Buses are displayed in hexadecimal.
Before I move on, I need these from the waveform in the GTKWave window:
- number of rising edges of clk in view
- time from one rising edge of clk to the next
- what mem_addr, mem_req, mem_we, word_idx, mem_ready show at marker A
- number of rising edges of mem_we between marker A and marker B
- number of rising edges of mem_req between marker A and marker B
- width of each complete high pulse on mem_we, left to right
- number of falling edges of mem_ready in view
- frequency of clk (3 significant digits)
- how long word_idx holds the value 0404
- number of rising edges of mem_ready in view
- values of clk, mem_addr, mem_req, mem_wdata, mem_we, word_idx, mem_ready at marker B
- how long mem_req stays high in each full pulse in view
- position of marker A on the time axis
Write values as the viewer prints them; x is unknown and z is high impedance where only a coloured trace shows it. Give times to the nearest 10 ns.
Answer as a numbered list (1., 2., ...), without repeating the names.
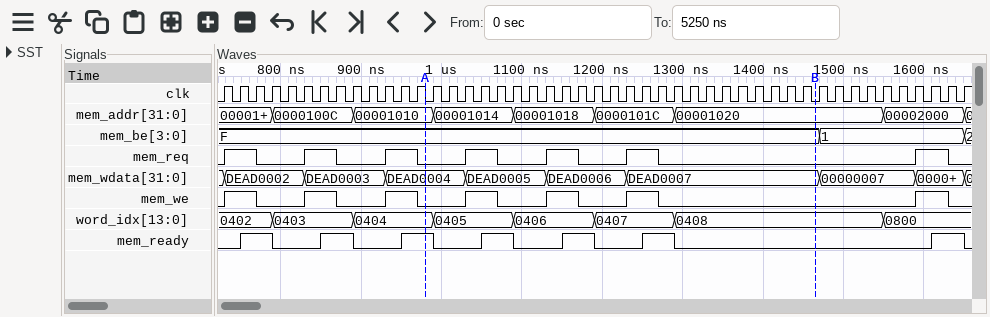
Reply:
1. 47
2. 20 ns
3. mem_addr=00001010, mem_req=0, mem_we=0, word_idx=0404, mem_ready=1
4. 3
5. 3
6. 40 ns, 40 ns, 40 ns, 40 ns, 40 ns, 40 ns, 40 ns
7. 7
8. 50.0 MHz
9. 100 ns
10. 7
11. clk=0, mem_addr=00001020, mem_req=0, mem_wdata=DEAD0007, mem_we=0, word_idx=0408, mem_ready=0
12. 40 ns, 40 ns, 40 ns, 40 ns, 40 ns, 40 ns, 40 ns
13. 980 ns
